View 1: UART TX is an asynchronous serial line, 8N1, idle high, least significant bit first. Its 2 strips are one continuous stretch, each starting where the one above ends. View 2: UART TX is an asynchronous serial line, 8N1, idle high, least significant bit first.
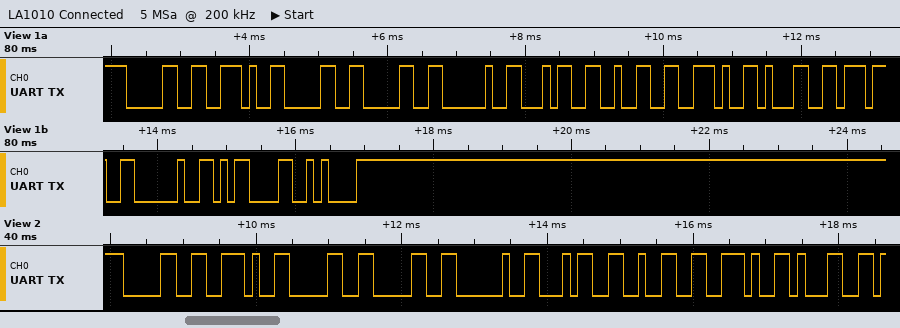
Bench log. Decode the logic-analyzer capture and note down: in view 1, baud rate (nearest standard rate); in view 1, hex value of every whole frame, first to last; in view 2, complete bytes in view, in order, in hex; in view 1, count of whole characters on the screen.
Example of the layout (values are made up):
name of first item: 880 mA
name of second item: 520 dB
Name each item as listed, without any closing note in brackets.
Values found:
in view 1, baud rate: 9600 baud
in view 1, hex value of every whole frame, first to last: 0x30 0x2E 0x30 0x30 0x20 0x34 0x32 0x2E 0x31 0x37 0x20 0x0D 0x0A
in view 2, complete bytes in view, in order, in hex: 30 2E 30 30 20 34 32 2E 31
in view 1, count of whole characters on the screen: 13
